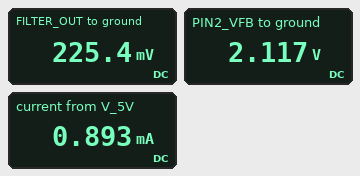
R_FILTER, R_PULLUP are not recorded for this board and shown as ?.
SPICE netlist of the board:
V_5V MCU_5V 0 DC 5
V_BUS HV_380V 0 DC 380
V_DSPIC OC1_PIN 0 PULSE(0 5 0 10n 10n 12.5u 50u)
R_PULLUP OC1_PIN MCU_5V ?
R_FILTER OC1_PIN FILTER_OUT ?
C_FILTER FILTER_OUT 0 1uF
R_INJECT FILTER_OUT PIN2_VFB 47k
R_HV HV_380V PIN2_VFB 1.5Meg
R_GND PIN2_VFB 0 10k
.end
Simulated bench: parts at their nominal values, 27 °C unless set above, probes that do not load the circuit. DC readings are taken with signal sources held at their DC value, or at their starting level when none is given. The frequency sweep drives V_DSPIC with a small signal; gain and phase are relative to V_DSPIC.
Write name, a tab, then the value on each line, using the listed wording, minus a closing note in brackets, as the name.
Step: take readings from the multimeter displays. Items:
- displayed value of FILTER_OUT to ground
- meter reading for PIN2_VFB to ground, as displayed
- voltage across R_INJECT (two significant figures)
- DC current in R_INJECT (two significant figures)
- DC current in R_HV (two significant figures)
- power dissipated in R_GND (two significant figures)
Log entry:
displayed value of FILTER_OUT to ground	225.4 mV
meter reading for PIN2_VFB to ground, as displayed	2.117 V
voltage across R_INJECT	1.9 V
DC current in R_INJECT	40 µA
DC current in R_HV	250 µA
power dissipated in R_GND	450 µW
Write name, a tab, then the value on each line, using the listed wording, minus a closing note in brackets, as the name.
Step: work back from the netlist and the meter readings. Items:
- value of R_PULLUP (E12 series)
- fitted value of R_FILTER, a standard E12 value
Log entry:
value of R_PULLUP	5.6 kΩ
fitted value of R_FILTER, a standard E12 value	5.6 kΩ
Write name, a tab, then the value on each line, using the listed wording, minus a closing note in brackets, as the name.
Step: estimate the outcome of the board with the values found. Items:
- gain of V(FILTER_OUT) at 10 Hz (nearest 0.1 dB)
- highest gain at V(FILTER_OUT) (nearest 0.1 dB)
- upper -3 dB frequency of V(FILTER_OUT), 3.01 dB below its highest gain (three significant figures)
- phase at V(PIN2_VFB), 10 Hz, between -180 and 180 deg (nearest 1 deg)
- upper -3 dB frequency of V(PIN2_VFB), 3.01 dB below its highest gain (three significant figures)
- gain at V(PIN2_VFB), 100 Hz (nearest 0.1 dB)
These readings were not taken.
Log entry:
gain of V(FILTER_OUT) at 10 Hz	-1.2 dB
highest gain at V(FILTER_OUT)	-0.8 dB
upper -3 dB frequency of V(FILTER_OUT), 3.01 dB below its highest gain	31.2 Hz
phase at V(PIN2_VFB), 10 Hz, between -180 and 180 deg	-18 deg
upper -3 dB frequency of V(PIN2_VFB), 3.01 dB below its highest gain	31.2 Hz
gain at V(PIN2_VFB), 100 Hz	-26.5 dB
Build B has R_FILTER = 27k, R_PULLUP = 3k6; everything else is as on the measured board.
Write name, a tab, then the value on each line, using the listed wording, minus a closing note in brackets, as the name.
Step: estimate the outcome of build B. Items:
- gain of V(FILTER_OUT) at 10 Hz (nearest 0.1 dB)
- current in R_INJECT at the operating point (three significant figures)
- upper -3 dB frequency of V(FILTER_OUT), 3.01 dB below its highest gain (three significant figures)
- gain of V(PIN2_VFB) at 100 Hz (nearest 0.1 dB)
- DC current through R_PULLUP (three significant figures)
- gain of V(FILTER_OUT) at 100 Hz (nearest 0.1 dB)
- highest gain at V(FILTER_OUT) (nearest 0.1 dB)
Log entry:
gain of V(FILTER_OUT) at 10 Hz	-7.0 dB
current in R_INJECT at the operating point	30.0 µA
upper -3 dB frequency of V(FILTER_OUT), 3.01 dB below its highest gain	8.69 Hz
gain of V(PIN2_VFB) at 100 Hz	-39.8 dB
DC current through R_PULLUP	1.39 mA
gain of V(FILTER_OUT) at 100 Hz	-24.6 dB
highest gain at V(FILTER_OUT)	-3.4 dB
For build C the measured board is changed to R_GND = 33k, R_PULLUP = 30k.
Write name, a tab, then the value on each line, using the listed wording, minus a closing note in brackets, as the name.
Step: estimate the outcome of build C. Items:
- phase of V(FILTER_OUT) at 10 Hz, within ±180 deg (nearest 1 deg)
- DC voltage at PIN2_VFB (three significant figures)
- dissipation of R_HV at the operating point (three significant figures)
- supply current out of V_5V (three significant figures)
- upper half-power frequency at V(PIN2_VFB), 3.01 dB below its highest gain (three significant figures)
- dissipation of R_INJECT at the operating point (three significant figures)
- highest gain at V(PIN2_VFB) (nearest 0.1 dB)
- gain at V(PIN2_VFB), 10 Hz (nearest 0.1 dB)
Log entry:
phase of V(FILTER_OUT) at 10 Hz, within ±180 deg	-18 deg
DC voltage at PIN2_VFB	5.07 V
dissipation of R_HV at the operating point	93.7 mW
supply current out of V_5V	167 µA
upper half-power frequency at V(PIN2_VFB), 3.01 dB below its highest gain	30.4 Hz
dissipation of R_INJECT at the operating point	436 µW
highest gain at V(PIN2_VFB)	-8.4 dB
gain at V(PIN2_VFB), 10 Hz	-8.8 dB
